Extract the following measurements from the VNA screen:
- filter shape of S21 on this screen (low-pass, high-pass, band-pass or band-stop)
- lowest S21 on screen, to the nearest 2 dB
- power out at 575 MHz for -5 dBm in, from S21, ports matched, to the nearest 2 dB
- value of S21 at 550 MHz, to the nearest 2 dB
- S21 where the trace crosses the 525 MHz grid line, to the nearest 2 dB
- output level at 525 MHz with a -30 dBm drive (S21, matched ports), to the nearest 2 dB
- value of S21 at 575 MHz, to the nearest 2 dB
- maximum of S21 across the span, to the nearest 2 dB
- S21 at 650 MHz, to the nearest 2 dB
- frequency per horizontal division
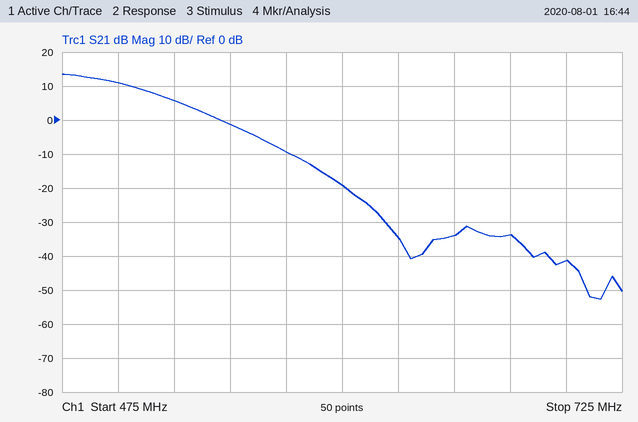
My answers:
low-pass
-52 dB
-14 dBm
-2 dB
6 dB
-24 dBm
-10 dB
14 dB
-34 dB
25 MHz
